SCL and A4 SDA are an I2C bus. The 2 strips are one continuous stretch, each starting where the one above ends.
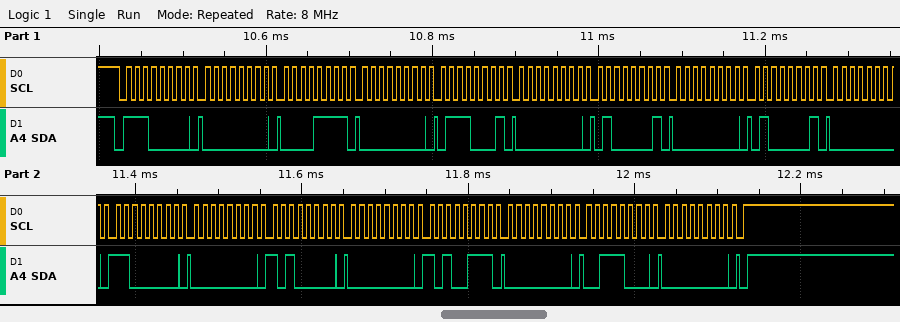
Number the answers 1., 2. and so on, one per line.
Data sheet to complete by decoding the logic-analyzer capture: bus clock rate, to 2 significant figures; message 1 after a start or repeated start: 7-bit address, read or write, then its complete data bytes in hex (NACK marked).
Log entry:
1. 100 kHz
2. 0x70 write: 00 0F 00 71 00 41 00 41 00 C0 00 A0 00 A7 00 38 00
